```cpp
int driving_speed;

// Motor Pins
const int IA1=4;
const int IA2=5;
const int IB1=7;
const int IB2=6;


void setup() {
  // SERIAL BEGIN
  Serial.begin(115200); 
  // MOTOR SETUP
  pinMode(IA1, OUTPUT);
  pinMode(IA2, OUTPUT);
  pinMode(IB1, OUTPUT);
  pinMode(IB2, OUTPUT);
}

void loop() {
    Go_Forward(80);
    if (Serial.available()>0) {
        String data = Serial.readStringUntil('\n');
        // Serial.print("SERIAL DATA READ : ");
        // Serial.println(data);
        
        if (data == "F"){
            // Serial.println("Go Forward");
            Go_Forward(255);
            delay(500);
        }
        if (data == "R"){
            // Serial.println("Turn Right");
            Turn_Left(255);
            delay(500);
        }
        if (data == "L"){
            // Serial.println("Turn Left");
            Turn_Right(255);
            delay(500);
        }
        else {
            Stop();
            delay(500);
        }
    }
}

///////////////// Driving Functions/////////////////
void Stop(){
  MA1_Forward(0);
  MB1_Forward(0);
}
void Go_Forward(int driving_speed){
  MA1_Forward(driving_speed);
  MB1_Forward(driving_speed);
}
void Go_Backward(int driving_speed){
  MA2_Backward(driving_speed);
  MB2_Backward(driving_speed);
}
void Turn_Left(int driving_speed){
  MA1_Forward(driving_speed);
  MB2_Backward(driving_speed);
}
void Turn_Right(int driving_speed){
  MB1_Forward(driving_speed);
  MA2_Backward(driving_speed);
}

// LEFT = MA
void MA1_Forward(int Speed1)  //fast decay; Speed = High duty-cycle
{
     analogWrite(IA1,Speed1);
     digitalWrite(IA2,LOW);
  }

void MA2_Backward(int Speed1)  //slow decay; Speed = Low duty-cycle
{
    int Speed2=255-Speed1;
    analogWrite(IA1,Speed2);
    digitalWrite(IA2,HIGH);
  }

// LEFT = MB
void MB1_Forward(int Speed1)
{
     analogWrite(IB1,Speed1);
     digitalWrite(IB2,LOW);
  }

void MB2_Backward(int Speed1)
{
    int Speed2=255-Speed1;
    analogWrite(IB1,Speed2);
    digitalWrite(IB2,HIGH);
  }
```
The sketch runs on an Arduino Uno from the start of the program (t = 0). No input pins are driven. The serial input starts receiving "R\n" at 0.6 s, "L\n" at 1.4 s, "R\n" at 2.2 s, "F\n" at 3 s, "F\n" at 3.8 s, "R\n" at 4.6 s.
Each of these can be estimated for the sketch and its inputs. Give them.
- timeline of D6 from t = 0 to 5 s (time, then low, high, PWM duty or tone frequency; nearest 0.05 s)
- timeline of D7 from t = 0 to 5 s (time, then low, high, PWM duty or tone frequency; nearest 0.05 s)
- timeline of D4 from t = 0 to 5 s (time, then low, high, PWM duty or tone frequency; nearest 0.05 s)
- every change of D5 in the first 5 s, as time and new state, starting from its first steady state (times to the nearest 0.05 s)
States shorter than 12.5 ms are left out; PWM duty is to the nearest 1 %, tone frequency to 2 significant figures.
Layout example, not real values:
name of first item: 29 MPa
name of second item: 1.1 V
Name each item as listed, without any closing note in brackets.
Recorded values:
timeline of D6 from t = 0 to 5 s: 0 s low; 0.6 s high; 1.1 s low; 2.2 s high; 2.7 s low
timeline of D7 from t = 0 to 5 s: 0 s low; 1.6 s high; 2.1 s low; 3.2 s high; 3.7 s low; 4.2 s high; 4.7 s low
timeline of D4 from t = 0 to 5 s: 0 s low; 0.6 s high; 1.1 s low; 2.2 s high; 2.7 s low; 3.2 s high; 3.7 s low; 4.2 s high; 4.7 s low
every change of D5 in the first 5 s, as time and new state, starting from its first steady state: 0 s low; 1.6 s high; 2.1 s low
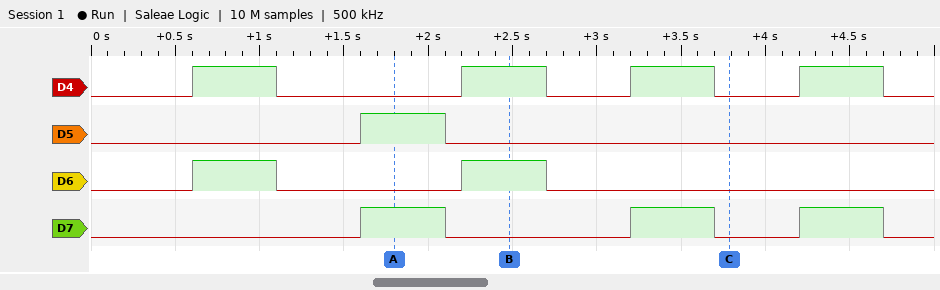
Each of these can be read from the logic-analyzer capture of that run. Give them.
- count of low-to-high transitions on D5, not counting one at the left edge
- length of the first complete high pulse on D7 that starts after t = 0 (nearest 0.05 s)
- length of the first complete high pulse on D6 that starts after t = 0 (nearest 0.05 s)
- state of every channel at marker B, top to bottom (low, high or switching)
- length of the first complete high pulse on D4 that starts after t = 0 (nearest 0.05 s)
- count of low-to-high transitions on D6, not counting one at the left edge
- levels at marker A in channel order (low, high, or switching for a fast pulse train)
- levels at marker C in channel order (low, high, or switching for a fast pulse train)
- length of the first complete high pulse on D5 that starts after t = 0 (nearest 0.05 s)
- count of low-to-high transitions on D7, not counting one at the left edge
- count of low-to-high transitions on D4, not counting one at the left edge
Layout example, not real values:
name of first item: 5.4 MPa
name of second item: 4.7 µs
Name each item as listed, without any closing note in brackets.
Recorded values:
count of low-to-high transitions on D5, not counting one at the left edge: 1
length of the first complete high pulse on D7 that starts after t = 0: 0.50 s
length of the first complete high pulse on D6 that starts after t = 0: 0.50 s
state of every channel at marker B, top to bottom: D4 high, D5 low, D6 high, D7 low
length of the first complete high pulse on D4 that starts after t = 0: 0.50 s
count of low-to-high transitions on D6, not counting one at the left edge: 2
levels at marker A in channel order: D4 low, D5 high, D6 low, D7 high
levels at marker C in channel order: D4 low, D5 low, D6 low, D7 low
length of the first complete high pulse on D5 that starts after t = 0: 0.50 s
count of low-to-high transitions on D7, not counting one at the left edge: 3
count of low-to-high transitions on D4, not counting one at the left edge: 4
